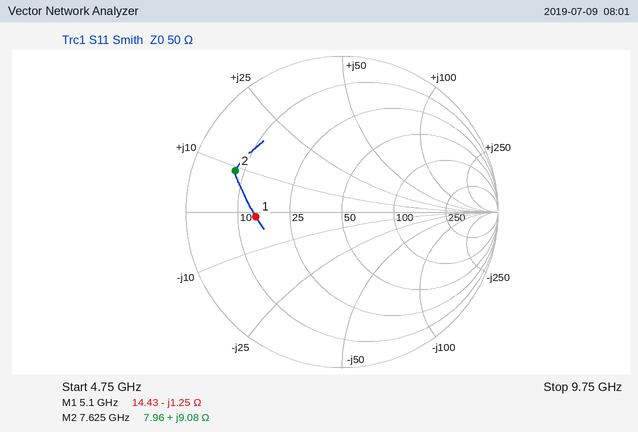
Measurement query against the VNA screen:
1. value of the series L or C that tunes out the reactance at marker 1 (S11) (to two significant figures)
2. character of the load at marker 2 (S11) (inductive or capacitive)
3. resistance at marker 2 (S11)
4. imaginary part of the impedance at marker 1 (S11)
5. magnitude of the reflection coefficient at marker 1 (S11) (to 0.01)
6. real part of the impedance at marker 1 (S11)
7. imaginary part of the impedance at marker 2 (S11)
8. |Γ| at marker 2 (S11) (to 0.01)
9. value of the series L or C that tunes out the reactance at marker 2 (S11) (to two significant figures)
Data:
39 pH
inductive
7.96 Ω
-1.25 Ω
0.55
14.43 Ω
+9.08 Ω
0.73
2.3 pF
